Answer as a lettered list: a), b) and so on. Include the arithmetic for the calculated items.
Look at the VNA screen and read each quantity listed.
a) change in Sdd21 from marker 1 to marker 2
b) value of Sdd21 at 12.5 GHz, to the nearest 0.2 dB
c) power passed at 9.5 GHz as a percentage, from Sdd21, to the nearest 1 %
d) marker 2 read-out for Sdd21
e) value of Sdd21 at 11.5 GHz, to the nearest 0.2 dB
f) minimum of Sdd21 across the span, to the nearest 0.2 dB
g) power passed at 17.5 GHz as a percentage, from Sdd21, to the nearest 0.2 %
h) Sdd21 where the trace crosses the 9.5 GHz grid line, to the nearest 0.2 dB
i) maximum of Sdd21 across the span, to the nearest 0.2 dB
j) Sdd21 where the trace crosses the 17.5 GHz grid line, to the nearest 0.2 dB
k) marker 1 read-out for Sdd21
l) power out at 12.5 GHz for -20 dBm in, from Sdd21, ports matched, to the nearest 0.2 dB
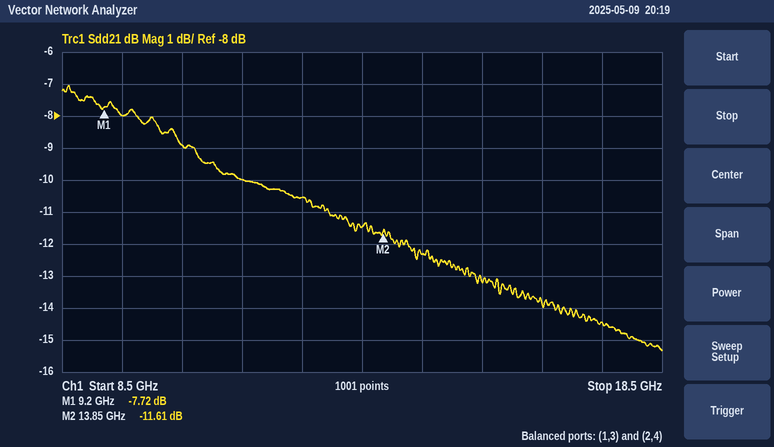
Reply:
a) -11.61 − (-7.72) = -3.89 dB
b) -10.6 dB
c) 10^(-8/10) ≈ 16 %
d) -11.61 dB
e) -10.0 dB
f) -15.4 dB
g) 10^(-14.4/10) ≈ 3.6 %
h) -8.0 dB
i) -7.0 dB
j) -14.4 dB
k) -7.72 dB
l) -20 dBm + (-10.6 dB) = -30.6 dBm
